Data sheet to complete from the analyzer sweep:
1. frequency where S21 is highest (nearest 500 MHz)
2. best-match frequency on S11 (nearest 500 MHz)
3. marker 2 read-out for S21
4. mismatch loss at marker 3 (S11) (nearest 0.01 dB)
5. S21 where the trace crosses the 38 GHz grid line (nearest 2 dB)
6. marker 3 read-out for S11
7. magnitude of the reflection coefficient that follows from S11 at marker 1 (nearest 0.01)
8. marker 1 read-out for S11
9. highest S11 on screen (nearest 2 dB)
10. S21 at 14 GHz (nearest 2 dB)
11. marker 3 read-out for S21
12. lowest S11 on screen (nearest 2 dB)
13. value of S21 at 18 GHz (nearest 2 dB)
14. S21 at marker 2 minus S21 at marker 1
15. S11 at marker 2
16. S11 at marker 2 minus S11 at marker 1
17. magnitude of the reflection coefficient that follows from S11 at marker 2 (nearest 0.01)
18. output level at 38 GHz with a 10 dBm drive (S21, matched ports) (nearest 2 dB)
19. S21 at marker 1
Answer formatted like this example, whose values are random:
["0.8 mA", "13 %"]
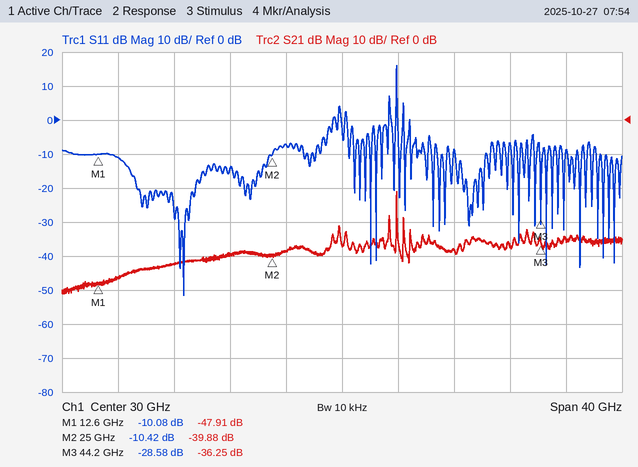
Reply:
["34.0 GHz", "18.5 GHz", "-39.88 dB", "0.01 dB", "-38 dB", "-28.58 dB", "0.31", "-10.08 dB", "16 dB", "-46 dB", "-36.25 dB", "-52 dB", "-42 dB", "8.03 dB", "-10.42 dB", "-0.34 dB", "0.30", "-28 dBm", "-47.91 dB"]
